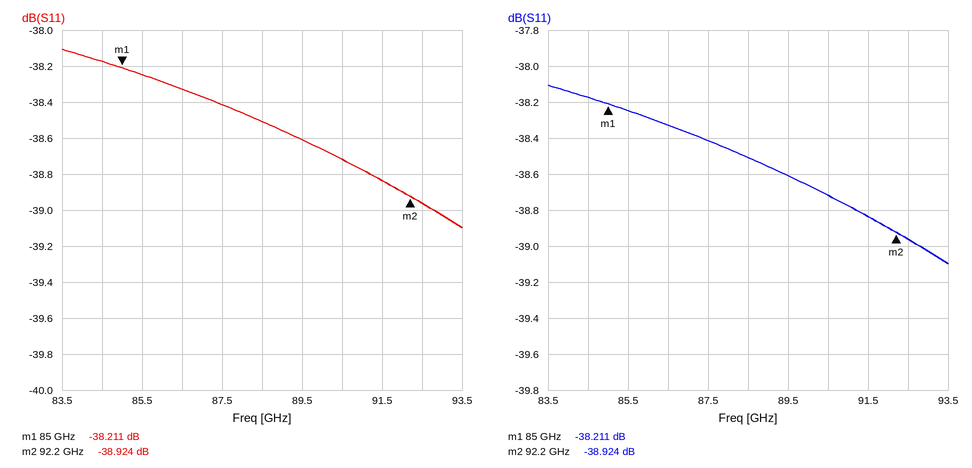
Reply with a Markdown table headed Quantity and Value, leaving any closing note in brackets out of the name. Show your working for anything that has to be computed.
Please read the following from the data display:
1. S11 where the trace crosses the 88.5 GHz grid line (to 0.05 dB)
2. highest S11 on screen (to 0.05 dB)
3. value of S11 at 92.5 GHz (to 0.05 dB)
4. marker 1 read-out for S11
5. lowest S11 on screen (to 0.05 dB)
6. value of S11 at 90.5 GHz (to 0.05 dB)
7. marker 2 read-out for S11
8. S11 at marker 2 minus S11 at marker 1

| Quantity | Value |
|---|---|
| S11 where the trace crosses the 88.5 GHz grid line | -38.50 dB |
| highest S11 on screen | -38.10 dB |
| value of S11 at 92.5 GHz | -38.95 dB |
| marker 1 read-out for S11 | -38.211 dB |
| lowest S11 on screen | -39.10 dB |
| value of S11 at 90.5 GHz | -38.70 dB |
| marker 2 read-out for S11 | -38.924 dB |
| S11 at marker 2 minus S11 at marker 1 | -38.924 − (-38.211) = -0.713 dB |
